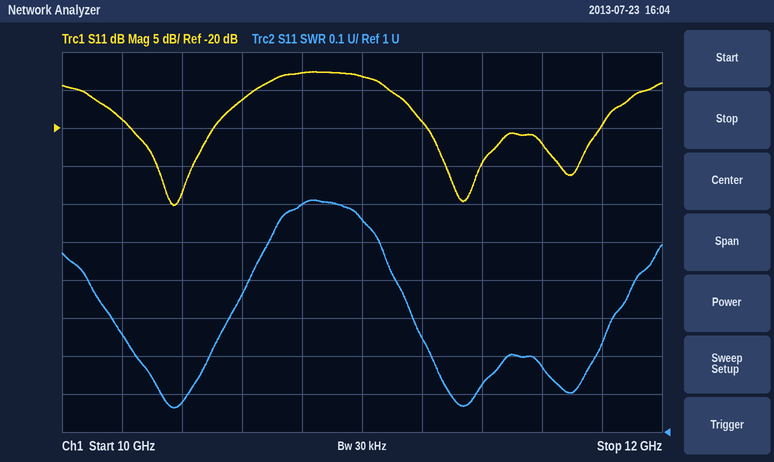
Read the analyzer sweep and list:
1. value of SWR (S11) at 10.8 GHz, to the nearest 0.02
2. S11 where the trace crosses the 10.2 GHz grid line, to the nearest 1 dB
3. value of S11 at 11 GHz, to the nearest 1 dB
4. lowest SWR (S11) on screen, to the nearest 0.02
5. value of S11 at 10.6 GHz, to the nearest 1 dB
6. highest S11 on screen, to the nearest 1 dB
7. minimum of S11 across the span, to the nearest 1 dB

1.60
-19 dB
-13 dB
1.06
-16 dB
-13 dB
-30 dB
